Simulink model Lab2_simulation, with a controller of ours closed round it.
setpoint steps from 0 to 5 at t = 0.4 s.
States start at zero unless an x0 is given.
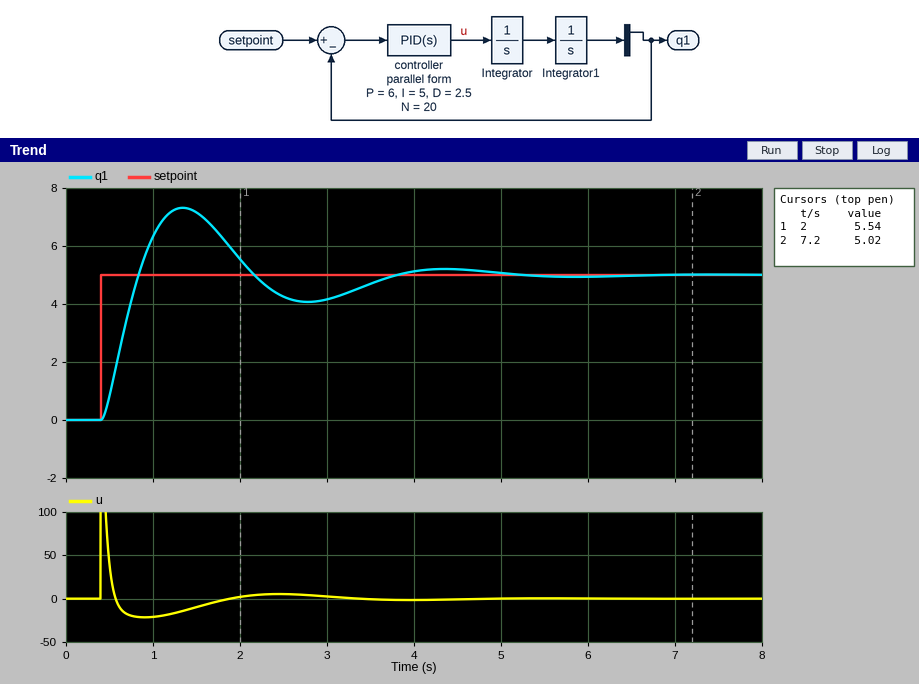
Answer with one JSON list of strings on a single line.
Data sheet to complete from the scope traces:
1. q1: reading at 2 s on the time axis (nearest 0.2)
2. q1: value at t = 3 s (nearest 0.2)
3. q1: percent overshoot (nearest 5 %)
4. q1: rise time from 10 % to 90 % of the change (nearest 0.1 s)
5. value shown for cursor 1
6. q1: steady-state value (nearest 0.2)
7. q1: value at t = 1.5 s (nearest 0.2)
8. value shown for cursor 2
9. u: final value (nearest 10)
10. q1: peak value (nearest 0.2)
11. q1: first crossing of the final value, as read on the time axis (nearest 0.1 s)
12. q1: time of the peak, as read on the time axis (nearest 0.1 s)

["5.6", "4.2", "45 %", "0.3 s", "5.54", "5.0", "7.2", "5.02", "0", "7.4", "0.8 s", "1.3 s"]
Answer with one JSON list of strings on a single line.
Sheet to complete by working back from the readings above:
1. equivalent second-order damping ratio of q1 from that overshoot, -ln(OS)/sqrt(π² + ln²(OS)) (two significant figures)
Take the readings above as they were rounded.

["0.25"]
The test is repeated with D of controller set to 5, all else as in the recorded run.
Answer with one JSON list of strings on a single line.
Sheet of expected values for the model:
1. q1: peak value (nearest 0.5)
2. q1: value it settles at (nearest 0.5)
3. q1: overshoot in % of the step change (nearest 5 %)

["6.0", "5.0", "20 %"]
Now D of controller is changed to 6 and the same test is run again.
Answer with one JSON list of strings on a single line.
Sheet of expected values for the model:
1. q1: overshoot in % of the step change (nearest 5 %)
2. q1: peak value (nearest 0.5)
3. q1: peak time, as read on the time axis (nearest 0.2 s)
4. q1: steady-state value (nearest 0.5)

["15 %", "6.0", "1.0 s", "5.0"]
